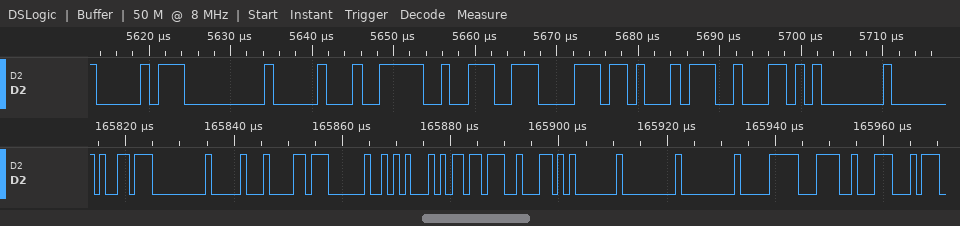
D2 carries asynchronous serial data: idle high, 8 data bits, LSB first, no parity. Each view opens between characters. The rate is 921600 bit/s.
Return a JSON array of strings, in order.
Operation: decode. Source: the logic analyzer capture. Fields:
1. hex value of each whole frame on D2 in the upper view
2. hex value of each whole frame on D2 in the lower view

["D0, 00, 10, 3E, CE, B8, D1, 62, 01", "D9, 00, 10, D8, 20, 45, DB, 62, 01, 00, 00, F0, 3C, 1C"]
